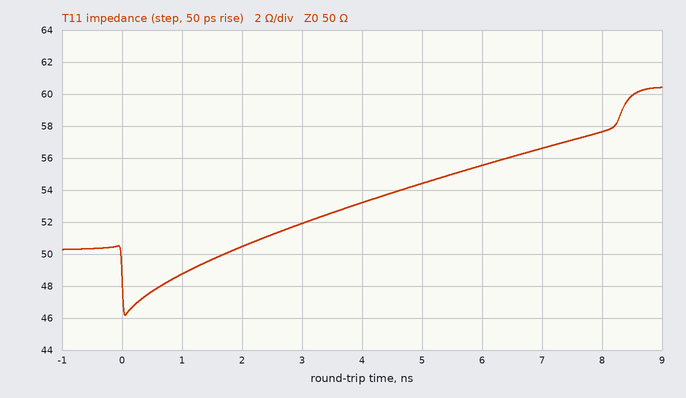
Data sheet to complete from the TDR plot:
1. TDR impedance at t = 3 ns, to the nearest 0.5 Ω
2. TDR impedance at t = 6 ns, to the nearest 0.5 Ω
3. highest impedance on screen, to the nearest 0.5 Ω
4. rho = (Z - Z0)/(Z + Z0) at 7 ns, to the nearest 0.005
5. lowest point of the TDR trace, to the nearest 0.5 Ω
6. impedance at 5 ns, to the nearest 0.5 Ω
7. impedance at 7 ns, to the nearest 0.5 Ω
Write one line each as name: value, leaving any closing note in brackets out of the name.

TDR impedance at t = 3 ns, to the nearest 0.5 Ω: 52.0 Ω
TDR impedance at t = 6 ns, to the nearest 0.5 Ω: 55.5 Ω
highest impedance on screen, to the nearest 0.5 Ω: 60.5 Ω
rho = (Z - Z0)/(Z + Z0) at 7 ns, to the nearest 0.005: +0.060
lowest point of the TDR trace, to the nearest 0.5 Ω: 46.0 Ω
impedance at 5 ns, to the nearest 0.5 Ω: 54.5 Ω
impedance at 7 ns, to the nearest 0.5 Ω: 56.5 Ω
